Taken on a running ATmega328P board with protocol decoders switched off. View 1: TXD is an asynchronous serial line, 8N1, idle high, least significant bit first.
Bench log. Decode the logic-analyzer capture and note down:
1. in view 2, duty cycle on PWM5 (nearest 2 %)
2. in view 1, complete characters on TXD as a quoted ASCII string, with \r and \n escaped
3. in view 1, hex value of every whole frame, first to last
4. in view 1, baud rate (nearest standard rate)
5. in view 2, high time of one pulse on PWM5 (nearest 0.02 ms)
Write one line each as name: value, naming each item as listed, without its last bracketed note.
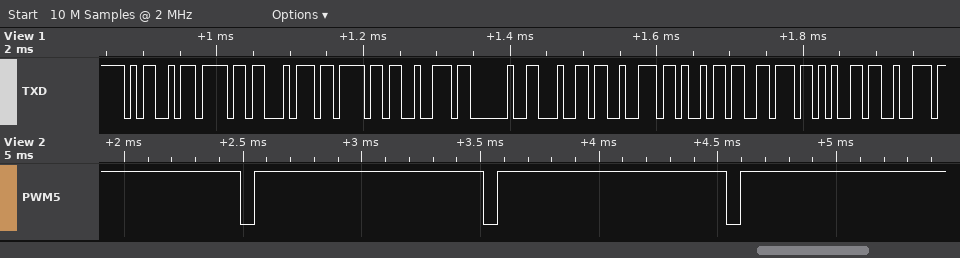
in view 2, duty cycle on PWM5: 94 %
in view 1, complete characters on TXD as a quoted ASCII string, with \r and \n escaped: "Motor driver"
in view 1, hex value of every whole frame, first to last: 0x4D 0x6F 0x74 0x6F 0x72 0x20 0x64 0x72 0x69 0x76 0x65 0x72
in view 1, baud rate: 115200 baud
in view 2, high time of one pulse on PWM5: 0.96 ms
